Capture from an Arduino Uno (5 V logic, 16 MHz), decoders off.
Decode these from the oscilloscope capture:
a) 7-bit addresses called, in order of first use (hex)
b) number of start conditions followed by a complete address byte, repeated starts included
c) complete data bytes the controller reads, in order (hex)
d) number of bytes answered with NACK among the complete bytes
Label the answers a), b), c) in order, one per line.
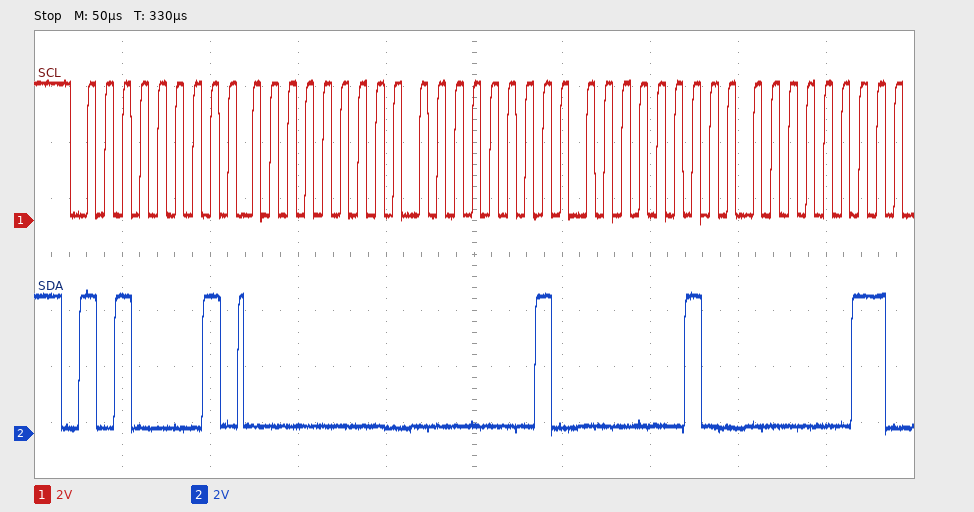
a) 0x50
b) 1
c) 00 01 02 03
d) 0
